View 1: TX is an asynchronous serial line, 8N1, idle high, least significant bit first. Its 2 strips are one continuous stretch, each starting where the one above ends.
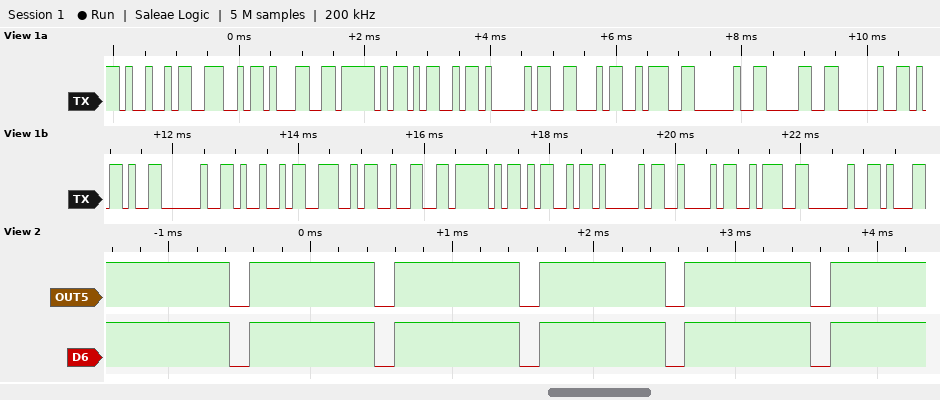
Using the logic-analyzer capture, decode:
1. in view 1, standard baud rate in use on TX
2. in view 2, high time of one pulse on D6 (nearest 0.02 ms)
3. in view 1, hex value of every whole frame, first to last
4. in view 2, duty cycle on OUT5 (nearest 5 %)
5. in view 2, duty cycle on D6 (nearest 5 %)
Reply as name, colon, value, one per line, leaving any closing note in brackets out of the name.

in view 1, standard baud rate in use on TX: 9600 baud
in view 2, high time of one pulse on D6: 0.88 ms
in view 1, hex value of every whole frame, first to last: 49 4E 31 5F 4D 41 46 3A 20 30 20 2D 20 49 4E 32 5F 4D 41 42 3A 20
in view 2, duty cycle on OUT5: 85 %
in view 2, duty cycle on D6: 85 %
